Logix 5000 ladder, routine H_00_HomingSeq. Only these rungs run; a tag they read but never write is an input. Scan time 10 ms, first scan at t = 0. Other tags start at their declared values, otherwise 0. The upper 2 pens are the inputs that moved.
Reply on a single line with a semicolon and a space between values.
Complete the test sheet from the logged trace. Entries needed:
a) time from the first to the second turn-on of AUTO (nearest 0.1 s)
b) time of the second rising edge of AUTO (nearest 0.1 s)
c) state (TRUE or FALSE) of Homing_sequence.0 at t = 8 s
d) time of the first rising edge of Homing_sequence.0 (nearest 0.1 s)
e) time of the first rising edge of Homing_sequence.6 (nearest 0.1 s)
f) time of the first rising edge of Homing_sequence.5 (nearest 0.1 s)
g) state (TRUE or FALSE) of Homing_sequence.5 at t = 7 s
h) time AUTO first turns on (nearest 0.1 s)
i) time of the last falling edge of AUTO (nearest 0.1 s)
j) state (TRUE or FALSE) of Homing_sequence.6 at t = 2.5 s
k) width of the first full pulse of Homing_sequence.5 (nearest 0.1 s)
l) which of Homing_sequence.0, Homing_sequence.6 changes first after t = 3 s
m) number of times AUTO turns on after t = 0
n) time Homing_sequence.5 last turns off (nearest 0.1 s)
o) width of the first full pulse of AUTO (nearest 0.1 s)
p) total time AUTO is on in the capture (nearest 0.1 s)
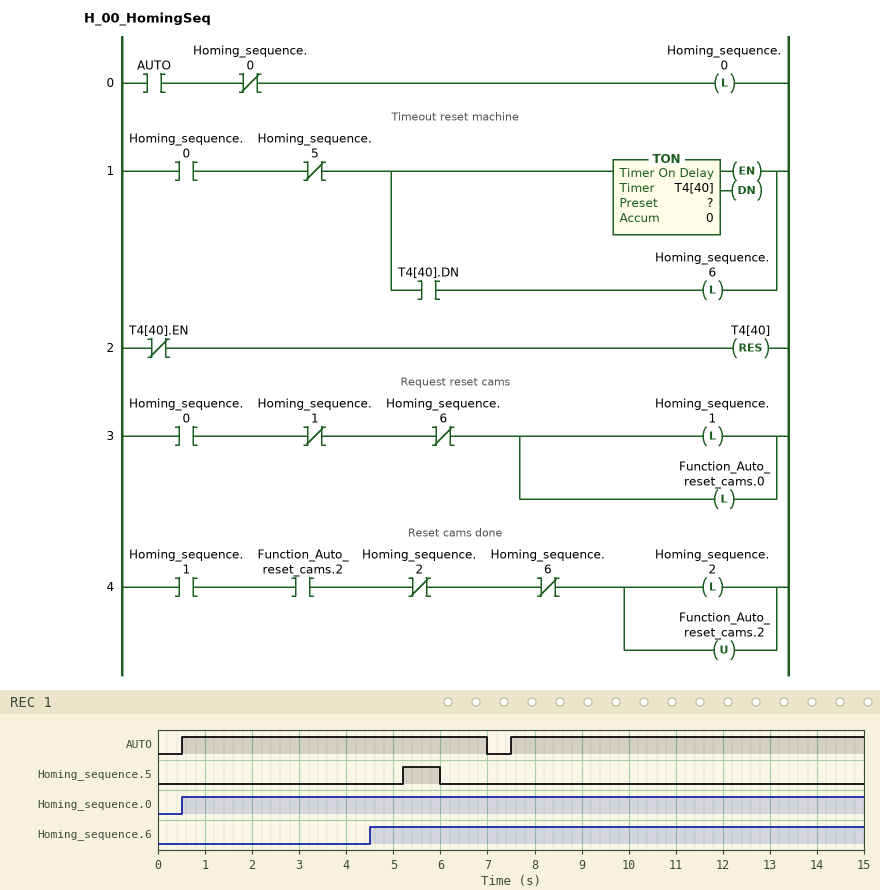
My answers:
7.0 s; 7.5 s; TRUE; 0.5 s; 4.5 s; 5.2 s; FALSE; 0.5 s; 7.0 s; FALSE; 0.8 s; Homing_sequence.6; 2; 6.0 s; 6.5 s; 14.0 s
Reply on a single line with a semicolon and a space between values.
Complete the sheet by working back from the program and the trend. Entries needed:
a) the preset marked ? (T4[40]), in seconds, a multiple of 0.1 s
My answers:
4.0 s
